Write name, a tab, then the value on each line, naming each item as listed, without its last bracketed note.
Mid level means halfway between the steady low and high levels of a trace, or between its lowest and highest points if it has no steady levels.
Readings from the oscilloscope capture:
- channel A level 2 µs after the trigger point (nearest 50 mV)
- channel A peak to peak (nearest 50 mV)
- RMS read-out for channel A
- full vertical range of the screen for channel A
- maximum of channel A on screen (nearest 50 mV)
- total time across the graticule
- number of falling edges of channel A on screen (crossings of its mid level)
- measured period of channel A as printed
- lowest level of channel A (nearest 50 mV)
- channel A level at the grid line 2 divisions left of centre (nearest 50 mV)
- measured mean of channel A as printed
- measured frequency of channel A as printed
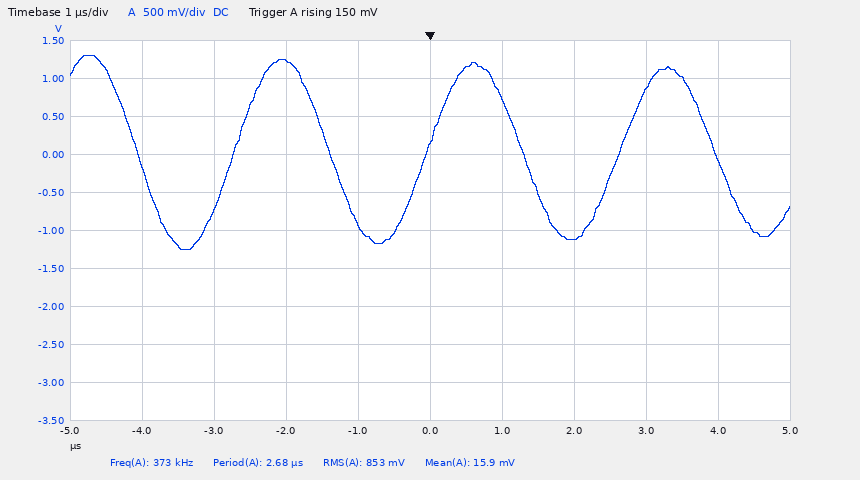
channel A level 2 µs after the trigger point	-1.10 V
channel A peak to peak	2.55 V
RMS read-out for channel A	853 mV
full vertical range of the screen for channel A	5 V
maximum of channel A on screen	1.30 V
total time across the graticule	10 µs
number of falling edges of channel A on screen	4
measured period of channel A as printed	2.68 µs
lowest level of channel A	-1.25 V
channel A level at the grid line 2 divisions left of centre	1.25 V
measured mean of channel A as printed	15.9 mV
measured frequency of channel A as printed	373 kHz
